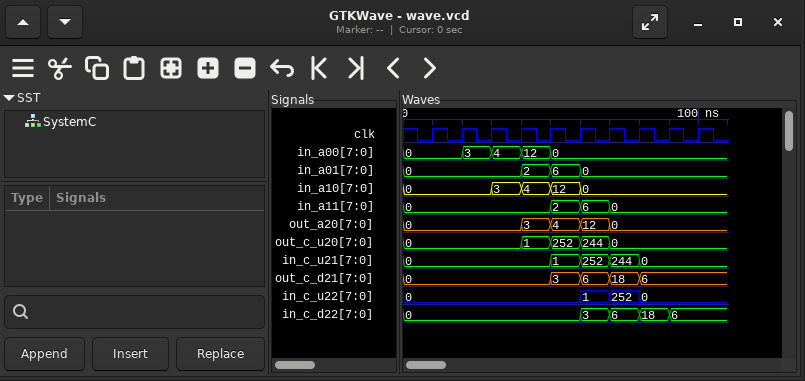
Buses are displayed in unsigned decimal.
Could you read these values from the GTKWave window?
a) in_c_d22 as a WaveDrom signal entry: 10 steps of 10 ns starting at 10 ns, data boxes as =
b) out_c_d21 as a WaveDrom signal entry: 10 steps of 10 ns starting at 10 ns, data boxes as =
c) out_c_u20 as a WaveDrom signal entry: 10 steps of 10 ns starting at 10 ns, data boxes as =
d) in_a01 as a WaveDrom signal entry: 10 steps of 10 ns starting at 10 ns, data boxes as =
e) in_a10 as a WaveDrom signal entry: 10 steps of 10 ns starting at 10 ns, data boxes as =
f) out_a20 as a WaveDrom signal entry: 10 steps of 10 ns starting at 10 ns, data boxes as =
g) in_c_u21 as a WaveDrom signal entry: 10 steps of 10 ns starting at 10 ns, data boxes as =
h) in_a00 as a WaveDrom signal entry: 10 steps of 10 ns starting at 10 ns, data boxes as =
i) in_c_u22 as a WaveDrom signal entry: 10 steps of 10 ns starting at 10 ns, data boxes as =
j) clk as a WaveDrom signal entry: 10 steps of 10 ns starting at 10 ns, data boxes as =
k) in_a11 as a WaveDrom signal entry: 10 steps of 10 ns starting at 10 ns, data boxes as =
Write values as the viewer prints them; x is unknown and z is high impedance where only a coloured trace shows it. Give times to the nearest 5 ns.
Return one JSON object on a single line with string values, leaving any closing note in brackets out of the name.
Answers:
{"in_c_d22 as a WaveDrom signal entry: 10 steps of 10 ns starting at 10 ns, data boxes as =": "{name: 'in_c_d22', wave: '=....====.', data: '0 3 6 18 6'}", "out_c_d21 as a WaveDrom signal entry: 10 steps of 10 ns starting at 10 ns, data boxes as =": "{name: 'out_c_d21', wave: '=...====..', data: '0 3 6 18 6'}", "out_c_u20 as a WaveDrom signal entry: 10 steps of 10 ns starting at 10 ns, data boxes as =": "{name: 'out_c_u20', wave: '=..====...', data: '0 1 252 244 0'}", "in_a01 as a WaveDrom signal entry: 10 steps of 10 ns starting at 10 ns, data boxes as =": "{name: 'in_a01', wave: '=..===....', data: '0 2 6 0'}", "in_a10 as a WaveDrom signal entry: 10 steps of 10 ns starting at 10 ns, data boxes as =": "{name: 'in_a10', wave: '=.====....', data: '0 3 4 12 0'}", "out_a20 as a WaveDrom signal entry: 10 steps of 10 ns starting at 10 ns, data boxes as =": "{name: 'out_a20', wave: '=..====...', data: '0 3 4 12 0'}", "in_c_u21 as a WaveDrom signal entry: 10 steps of 10 ns starting at 10 ns, data boxes as =": "{name: 'in_c_u21', wave: '=...====..', data: '0 1 252 244 0'}", "in_a00 as a WaveDrom signal entry: 10 steps of 10 ns starting at 10 ns, data boxes as =": "{name: 'in_a00', wave: '=====.....', data: '0 3 4 12 0'}", "in_c_u22 as a WaveDrom signal entry: 10 steps of 10 ns starting at 10 ns, data boxes as =": "{name: 'in_c_u22', wave: '=....===..', data: '0 1 252 0'}", "clk as a WaveDrom signal entry: 10 steps of 10 ns starting at 10 ns, data boxes as =": "{name: 'clk', wave: 'p.........'}", "in_a11 as a WaveDrom signal entry: 10 steps of 10 ns starting at 10 ns, data boxes as =": "{name: 'in_a11', wave: '=...===...', data: '0 2 6 0'}"}
